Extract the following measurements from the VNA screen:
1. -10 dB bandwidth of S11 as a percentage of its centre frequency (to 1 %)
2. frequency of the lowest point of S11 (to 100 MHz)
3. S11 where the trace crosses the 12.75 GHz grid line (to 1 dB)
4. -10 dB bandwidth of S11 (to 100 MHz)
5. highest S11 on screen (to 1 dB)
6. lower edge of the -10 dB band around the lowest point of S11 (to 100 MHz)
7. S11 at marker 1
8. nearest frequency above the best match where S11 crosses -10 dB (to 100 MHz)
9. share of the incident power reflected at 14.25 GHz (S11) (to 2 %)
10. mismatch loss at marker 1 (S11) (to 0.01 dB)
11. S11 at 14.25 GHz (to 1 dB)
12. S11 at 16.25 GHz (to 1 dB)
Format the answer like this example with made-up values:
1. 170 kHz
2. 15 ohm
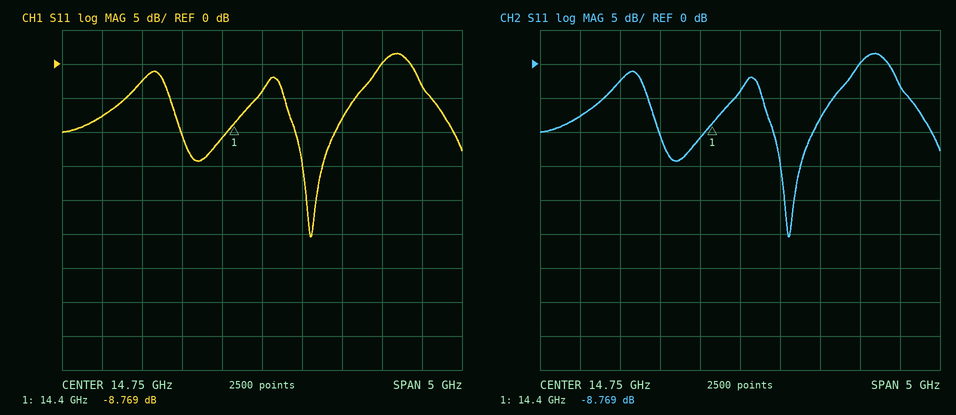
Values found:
1. 3 %
2. 15.4 GHz
3. -8 dB
4. 500 MHz
5. 2 dB
6. 15.2 GHz
7. -8.769 dB
8. 15.7 GHz
9. 8 %
10. 0.62 dB
11. -11 dB
12. 0 dB
